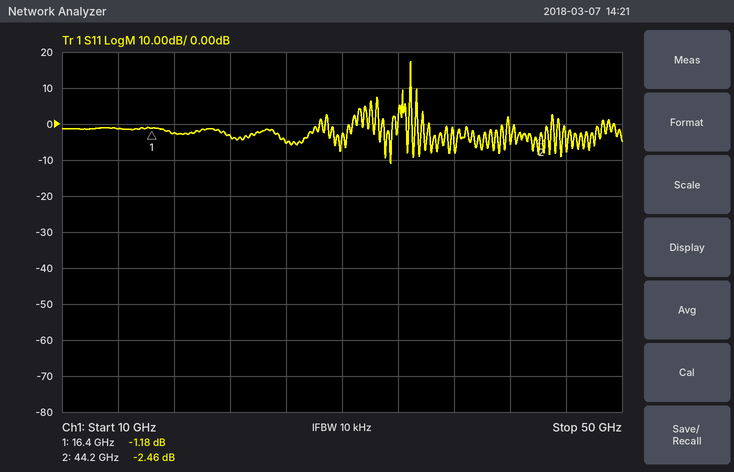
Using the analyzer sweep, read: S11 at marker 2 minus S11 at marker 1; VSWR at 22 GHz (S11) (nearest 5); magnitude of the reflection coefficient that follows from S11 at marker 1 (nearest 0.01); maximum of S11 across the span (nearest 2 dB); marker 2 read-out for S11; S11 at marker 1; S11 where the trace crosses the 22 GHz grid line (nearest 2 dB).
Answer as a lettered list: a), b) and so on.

a) -1.28 dB
b) 5
c) 0.87
d) 18 dB
e) -2.46 dB
f) -1.18 dB
g) -4 dB
